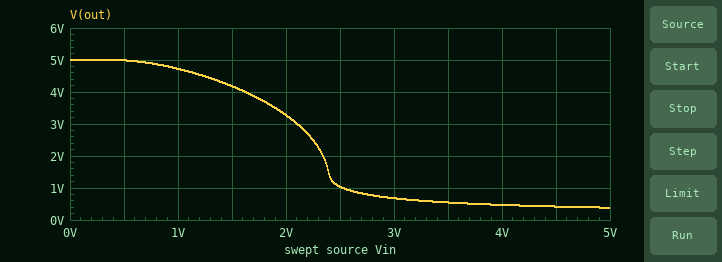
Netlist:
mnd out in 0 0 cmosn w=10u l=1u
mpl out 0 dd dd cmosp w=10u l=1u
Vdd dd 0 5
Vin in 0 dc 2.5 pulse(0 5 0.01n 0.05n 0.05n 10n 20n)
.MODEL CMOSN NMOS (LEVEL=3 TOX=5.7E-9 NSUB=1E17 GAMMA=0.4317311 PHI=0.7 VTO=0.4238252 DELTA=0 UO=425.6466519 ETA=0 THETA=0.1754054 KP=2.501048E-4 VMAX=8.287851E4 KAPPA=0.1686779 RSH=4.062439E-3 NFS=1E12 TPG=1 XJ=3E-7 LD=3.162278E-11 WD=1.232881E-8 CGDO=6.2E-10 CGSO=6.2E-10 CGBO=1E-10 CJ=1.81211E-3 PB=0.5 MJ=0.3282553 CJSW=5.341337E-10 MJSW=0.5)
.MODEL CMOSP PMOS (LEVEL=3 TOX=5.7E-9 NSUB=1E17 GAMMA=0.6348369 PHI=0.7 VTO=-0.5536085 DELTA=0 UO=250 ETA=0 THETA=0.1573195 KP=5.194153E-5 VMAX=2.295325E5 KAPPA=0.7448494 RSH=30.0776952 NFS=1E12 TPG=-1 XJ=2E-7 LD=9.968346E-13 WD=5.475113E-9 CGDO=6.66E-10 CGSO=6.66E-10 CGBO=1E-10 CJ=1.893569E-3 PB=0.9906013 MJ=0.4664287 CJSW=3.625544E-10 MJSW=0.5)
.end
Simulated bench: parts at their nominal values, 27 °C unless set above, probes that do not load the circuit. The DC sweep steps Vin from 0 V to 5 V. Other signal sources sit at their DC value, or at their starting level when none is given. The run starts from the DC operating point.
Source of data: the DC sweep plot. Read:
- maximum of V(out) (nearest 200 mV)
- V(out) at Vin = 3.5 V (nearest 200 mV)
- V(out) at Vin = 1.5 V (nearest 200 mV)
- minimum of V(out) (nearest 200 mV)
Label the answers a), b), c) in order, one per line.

a) 5.0 V
b) 600 mV
c) 4.2 V
d) 400 mV
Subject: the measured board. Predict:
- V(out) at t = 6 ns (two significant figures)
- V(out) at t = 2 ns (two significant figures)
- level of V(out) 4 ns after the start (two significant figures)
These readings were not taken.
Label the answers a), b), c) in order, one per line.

a) 380 mV
b) 380 mV
c) 380 mV
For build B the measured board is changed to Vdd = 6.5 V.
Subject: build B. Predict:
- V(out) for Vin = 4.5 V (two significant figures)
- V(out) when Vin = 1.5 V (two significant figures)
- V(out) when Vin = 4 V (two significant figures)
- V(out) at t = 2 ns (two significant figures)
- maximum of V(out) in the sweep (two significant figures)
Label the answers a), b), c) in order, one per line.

a) 720 mV
b) 5.8 V
c) 840 mV
d) 640 mV
e) 6.5 V
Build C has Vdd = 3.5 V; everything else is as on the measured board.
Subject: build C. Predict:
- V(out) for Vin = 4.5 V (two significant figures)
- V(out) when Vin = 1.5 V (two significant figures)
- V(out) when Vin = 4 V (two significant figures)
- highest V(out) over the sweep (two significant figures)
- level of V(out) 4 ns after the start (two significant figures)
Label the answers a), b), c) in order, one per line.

a) 210 mV
b) 2.3 V
c) 230 mV
d) 3.5 V
e) 190 mV
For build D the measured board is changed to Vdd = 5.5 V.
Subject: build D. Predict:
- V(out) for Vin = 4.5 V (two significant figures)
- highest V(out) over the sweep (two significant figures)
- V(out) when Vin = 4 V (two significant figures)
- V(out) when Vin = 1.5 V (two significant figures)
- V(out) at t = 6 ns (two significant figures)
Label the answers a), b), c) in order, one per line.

a) 510 mV
b) 5.5 V
c) 580 mV
d) 4.7 V
e) 460 mV
